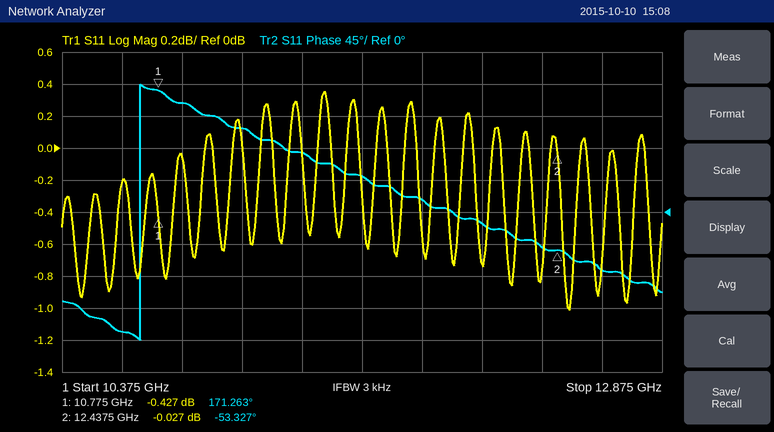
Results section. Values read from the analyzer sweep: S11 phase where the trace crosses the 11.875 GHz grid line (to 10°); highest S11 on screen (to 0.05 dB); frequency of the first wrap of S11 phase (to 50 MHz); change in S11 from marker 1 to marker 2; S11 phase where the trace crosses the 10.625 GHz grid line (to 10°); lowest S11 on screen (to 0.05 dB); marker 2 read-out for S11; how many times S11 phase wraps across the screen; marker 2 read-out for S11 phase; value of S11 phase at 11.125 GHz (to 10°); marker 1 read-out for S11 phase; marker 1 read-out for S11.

20°
0.35 dB
10.70 GHz
0.400 dB
-170°
-1.00 dB
-0.027 dB
1
-53.327°
120°
171.263°
-0.427 dB
